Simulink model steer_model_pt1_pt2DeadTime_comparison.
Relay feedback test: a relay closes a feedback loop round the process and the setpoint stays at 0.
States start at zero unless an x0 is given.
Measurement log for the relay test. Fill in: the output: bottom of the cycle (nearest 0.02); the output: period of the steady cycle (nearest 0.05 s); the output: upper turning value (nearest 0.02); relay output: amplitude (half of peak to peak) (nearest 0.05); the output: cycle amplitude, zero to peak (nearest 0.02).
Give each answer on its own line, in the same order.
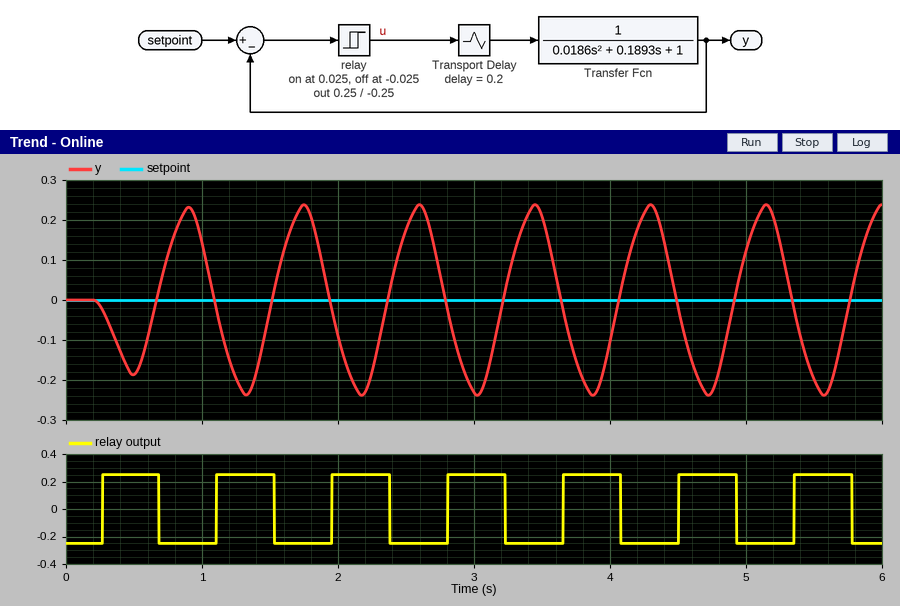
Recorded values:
-0.24
0.85 s
0.24
0.25
0.24
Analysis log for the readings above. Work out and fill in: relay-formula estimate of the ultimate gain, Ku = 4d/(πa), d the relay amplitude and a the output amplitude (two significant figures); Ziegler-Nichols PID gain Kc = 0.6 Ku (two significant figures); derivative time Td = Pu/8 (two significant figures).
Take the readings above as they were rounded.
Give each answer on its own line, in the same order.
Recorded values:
1.3
0.78
0.11 s
